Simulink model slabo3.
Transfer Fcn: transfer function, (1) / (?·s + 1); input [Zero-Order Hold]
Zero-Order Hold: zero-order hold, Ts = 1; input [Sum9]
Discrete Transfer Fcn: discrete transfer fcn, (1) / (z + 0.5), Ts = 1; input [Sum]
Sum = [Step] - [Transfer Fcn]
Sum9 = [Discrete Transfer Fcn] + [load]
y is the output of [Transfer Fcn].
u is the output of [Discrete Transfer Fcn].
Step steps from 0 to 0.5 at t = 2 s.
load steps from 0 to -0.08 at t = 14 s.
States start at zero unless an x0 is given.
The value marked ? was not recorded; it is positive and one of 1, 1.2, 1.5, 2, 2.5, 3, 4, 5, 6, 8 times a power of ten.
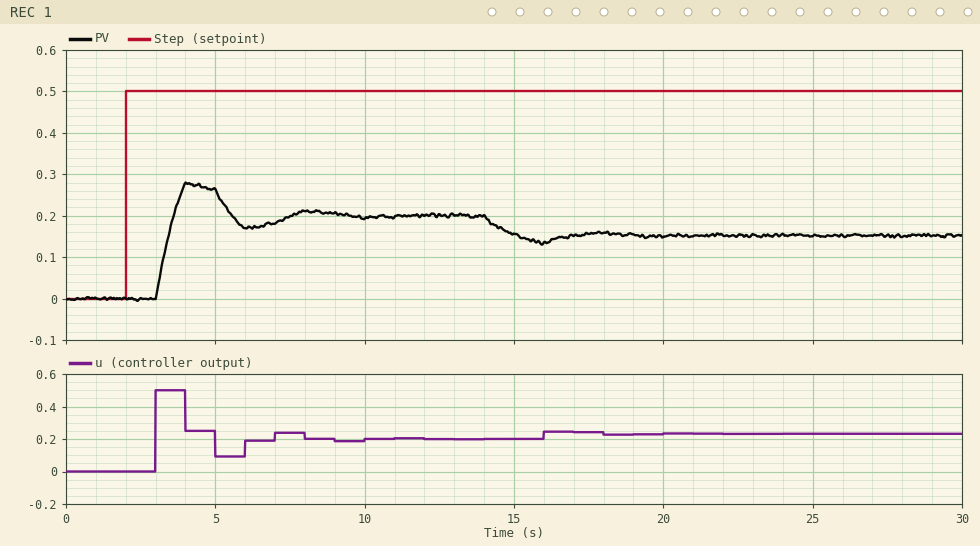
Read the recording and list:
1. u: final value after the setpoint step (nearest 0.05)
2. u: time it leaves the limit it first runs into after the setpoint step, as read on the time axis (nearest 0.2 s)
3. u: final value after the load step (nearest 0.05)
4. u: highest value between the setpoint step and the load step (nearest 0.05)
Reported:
0.20
3.0 s
0.25
0.50
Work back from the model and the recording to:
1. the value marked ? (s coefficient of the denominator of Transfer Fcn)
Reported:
1.2
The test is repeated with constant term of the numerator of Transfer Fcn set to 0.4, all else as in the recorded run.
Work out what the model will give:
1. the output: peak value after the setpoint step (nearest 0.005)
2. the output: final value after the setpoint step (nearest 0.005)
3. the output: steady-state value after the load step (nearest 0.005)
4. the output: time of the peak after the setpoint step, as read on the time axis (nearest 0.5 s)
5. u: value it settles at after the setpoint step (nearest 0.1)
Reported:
0.115
0.105
0.080
4.0 s
0.3
